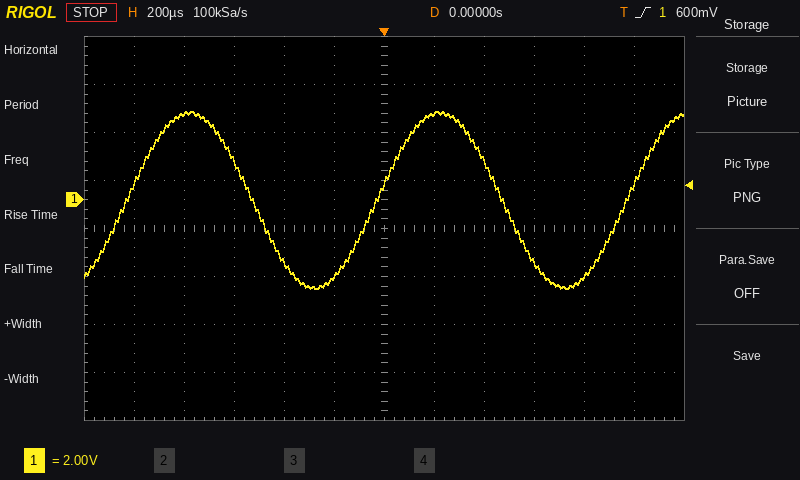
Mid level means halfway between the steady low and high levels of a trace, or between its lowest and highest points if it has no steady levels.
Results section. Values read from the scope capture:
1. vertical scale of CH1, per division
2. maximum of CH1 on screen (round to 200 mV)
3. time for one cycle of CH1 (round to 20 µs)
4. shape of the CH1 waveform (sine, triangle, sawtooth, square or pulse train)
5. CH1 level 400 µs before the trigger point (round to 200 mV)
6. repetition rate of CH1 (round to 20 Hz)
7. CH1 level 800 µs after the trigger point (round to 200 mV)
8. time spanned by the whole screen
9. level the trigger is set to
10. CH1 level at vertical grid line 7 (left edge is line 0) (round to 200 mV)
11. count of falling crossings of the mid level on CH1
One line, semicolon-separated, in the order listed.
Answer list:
2 V; 3.6 V; 1.00 ms; sine; -2.6 V; 1.00 kHz; -3.2 V; 2.4 ms; 600 mV; 3.6 V; 2
